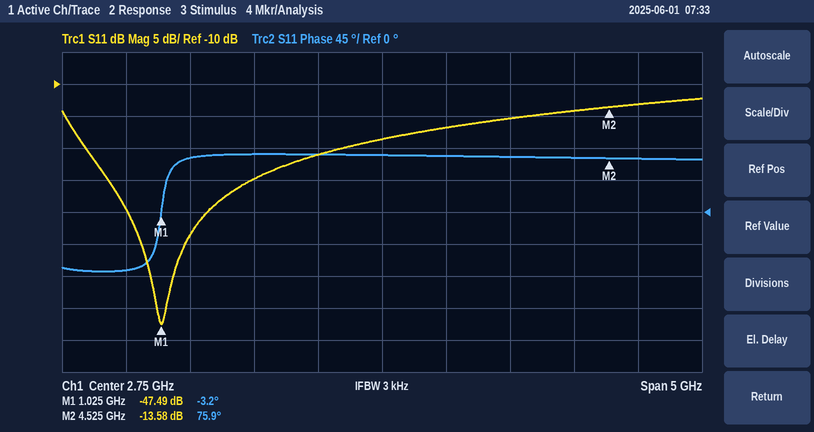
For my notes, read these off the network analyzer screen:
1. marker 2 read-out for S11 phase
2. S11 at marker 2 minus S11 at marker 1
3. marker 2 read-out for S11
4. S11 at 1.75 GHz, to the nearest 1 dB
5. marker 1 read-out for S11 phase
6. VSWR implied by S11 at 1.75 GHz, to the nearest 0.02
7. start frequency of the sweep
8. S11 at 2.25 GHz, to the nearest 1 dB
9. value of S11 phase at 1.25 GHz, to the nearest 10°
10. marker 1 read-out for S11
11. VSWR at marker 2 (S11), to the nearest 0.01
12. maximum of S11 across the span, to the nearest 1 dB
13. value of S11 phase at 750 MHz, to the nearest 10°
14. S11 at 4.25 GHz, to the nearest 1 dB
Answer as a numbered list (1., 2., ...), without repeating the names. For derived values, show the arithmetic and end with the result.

1. 75.9°
2. -13.58 − (-47.49) = 33.91 dB
3. -13.58 dB
4. -25 dB
5. -3.2°
6. |Γ| = 10^(-25/20) = 0.0562; VSWR = (1 + 0.0562)/(1 − 0.0562) ≈ 1.12
7. 250 MHz
8. -21 dB
9. 80°
10. -47.49 dB
11. (1 + 0.2094)/(1 − 0.2094) ≈ 1.53
12. -12 dB
13. -80°
14. -14 dB
